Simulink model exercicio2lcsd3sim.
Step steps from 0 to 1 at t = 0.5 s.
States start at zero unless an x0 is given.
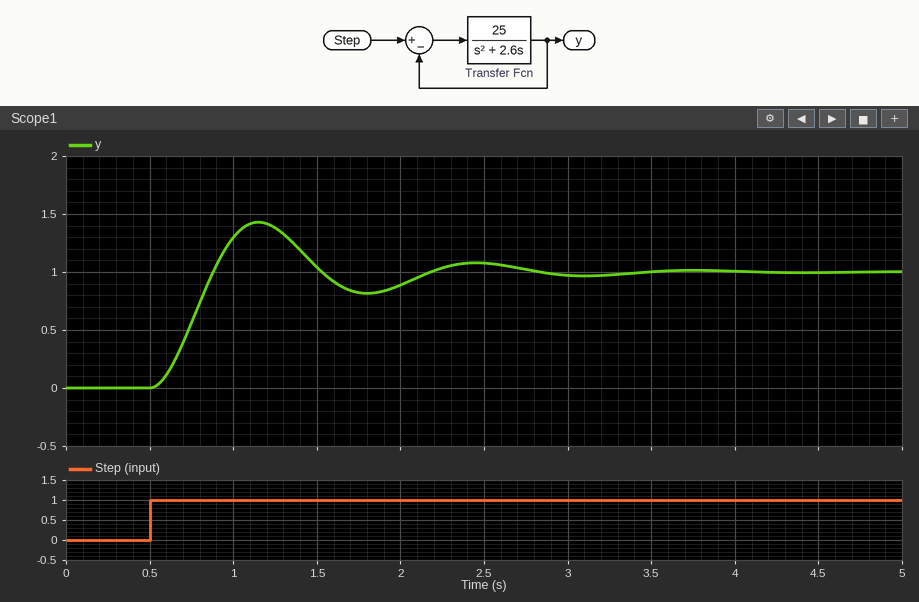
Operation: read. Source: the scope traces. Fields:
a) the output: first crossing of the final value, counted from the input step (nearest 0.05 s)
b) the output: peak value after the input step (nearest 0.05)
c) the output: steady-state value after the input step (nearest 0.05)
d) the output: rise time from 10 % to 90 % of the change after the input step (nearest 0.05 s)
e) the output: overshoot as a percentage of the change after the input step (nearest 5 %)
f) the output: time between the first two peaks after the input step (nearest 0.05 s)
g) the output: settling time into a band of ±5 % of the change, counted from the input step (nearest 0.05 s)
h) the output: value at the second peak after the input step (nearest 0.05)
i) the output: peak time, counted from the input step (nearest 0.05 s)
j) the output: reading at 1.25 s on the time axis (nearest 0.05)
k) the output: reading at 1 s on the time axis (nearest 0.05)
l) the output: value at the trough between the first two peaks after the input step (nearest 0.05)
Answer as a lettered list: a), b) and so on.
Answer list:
a) 0.40 s
b) 1.45
c) 1.00
d) 0.25 s
e) 45 %
f) 1.30 s
g) 2.15 s
h) 1.10
i) 0.65 s
j) 1.40
k) 1.30
l) 0.80
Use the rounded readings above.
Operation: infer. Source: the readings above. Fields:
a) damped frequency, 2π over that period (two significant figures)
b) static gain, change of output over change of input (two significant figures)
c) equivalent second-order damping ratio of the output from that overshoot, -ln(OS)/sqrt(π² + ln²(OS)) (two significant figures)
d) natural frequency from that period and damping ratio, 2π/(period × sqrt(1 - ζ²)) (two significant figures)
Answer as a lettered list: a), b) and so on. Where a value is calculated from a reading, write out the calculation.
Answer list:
a) 2π / 1.3 = 4.8 rad/s
b) (1 - 0) / (1 - 0) = 1.0
c) ln(0.45) = -0.799; 0.799 / sqrt(9.870 + 0.638) = 0.25
d) 2π / (1.3 × sqrt(1 - 0.25²)) = 5.0 rad/s
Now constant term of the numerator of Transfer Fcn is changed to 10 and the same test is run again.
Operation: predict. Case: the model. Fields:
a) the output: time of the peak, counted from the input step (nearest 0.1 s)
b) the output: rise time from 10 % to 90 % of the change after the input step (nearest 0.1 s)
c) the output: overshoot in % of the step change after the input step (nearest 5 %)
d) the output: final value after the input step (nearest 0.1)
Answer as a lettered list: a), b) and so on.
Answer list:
a) 1.1 s
b) 0.5 s
c) 25 %
d) 1.0
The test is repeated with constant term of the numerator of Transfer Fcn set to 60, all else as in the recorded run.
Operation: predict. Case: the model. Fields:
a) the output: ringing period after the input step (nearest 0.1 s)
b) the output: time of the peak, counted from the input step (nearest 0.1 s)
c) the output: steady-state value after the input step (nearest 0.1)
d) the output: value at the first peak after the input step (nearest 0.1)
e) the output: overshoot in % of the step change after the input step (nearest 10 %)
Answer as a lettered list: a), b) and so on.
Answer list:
a) 0.8 s
b) 0.4 s
c) 1.0
d) 1.6
e) 60 %
